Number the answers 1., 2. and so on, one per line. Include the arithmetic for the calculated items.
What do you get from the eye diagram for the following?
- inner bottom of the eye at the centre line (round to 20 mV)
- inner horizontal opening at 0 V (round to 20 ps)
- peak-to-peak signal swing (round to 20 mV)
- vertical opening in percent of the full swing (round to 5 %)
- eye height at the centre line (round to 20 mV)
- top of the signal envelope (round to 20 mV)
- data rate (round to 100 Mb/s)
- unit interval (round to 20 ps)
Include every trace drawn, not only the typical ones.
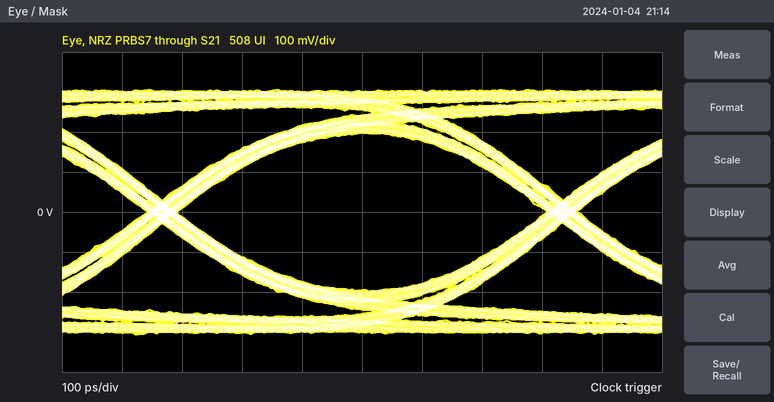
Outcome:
1. -200 mV
2. 620 ps
3. 620 mV
4. 400 mV / 620 mV ≈ 65 %
5. 400 mV
6. 300 mV
7. 1.5 Gb/s
8. 660 ps
